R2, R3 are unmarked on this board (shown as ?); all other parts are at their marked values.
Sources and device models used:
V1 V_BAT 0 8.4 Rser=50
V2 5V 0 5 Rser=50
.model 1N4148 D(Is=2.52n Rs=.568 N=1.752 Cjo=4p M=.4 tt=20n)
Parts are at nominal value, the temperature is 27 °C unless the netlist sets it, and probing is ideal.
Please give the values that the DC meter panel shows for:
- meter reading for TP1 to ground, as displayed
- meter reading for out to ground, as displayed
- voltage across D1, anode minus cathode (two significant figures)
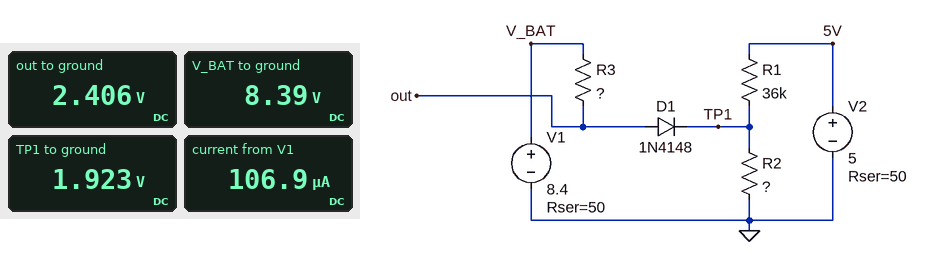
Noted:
1.923 V
2.406 V
480 mV
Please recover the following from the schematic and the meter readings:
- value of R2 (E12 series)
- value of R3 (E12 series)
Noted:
10 kΩ
56 kΩ
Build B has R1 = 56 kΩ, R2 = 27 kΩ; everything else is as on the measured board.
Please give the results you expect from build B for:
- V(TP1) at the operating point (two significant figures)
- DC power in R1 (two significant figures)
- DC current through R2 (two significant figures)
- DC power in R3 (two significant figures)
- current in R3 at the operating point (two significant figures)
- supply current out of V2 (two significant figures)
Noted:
3.2 V
60 µW
120 µA
400 µW
85 µA
33 µA
